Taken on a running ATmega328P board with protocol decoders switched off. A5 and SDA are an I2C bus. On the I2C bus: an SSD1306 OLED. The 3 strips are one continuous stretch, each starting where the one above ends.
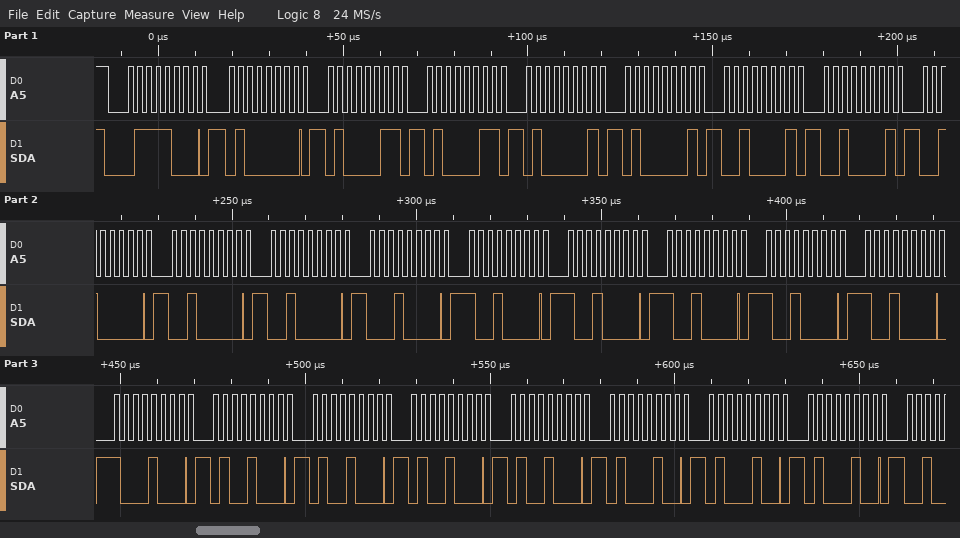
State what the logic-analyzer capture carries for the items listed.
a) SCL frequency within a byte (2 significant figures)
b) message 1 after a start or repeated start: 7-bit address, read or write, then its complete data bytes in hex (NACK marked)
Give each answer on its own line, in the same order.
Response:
400 kHz
0x3C write: 40 43 43 41 41 21 21 20 20 20 10 90 90 90 90 90 88 48 48 48 48 44 44 44
